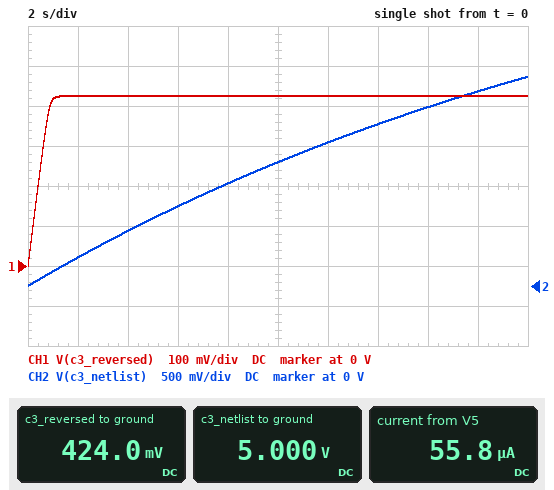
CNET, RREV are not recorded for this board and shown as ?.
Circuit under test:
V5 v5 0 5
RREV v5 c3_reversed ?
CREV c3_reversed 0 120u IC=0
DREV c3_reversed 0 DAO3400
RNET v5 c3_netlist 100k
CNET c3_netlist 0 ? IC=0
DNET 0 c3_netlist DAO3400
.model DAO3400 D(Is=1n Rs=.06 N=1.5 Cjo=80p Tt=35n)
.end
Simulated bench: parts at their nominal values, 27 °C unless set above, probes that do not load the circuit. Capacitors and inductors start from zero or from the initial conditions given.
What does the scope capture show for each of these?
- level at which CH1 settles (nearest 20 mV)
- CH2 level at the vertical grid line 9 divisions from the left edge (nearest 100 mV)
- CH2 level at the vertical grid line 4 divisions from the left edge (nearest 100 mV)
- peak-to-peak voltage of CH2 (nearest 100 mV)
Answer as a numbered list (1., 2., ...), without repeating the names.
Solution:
1. 420 mV
2. 2.4 V
3. 1.3 V
4. 2.6 V
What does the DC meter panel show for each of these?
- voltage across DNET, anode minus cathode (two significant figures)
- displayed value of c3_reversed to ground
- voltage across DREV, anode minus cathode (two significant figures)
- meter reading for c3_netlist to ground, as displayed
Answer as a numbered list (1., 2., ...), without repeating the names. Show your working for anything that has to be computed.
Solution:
1. 0 V - 5 V = -5.0 V
2. 424.0 mV
3. 424 mV = 420 mV
4. 5.000 V
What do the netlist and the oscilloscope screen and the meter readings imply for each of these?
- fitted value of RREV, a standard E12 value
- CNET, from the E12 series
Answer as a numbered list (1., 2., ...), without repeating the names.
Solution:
1. 82 kΩ
2. 270 µF
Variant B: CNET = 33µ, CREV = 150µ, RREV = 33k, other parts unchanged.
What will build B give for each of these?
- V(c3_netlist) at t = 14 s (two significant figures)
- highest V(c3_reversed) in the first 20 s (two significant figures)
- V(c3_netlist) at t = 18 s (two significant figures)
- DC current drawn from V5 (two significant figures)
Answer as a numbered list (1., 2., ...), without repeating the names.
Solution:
1. 4.9 V
2. 460 mV
3. 5.0 V
4. 140 µA
